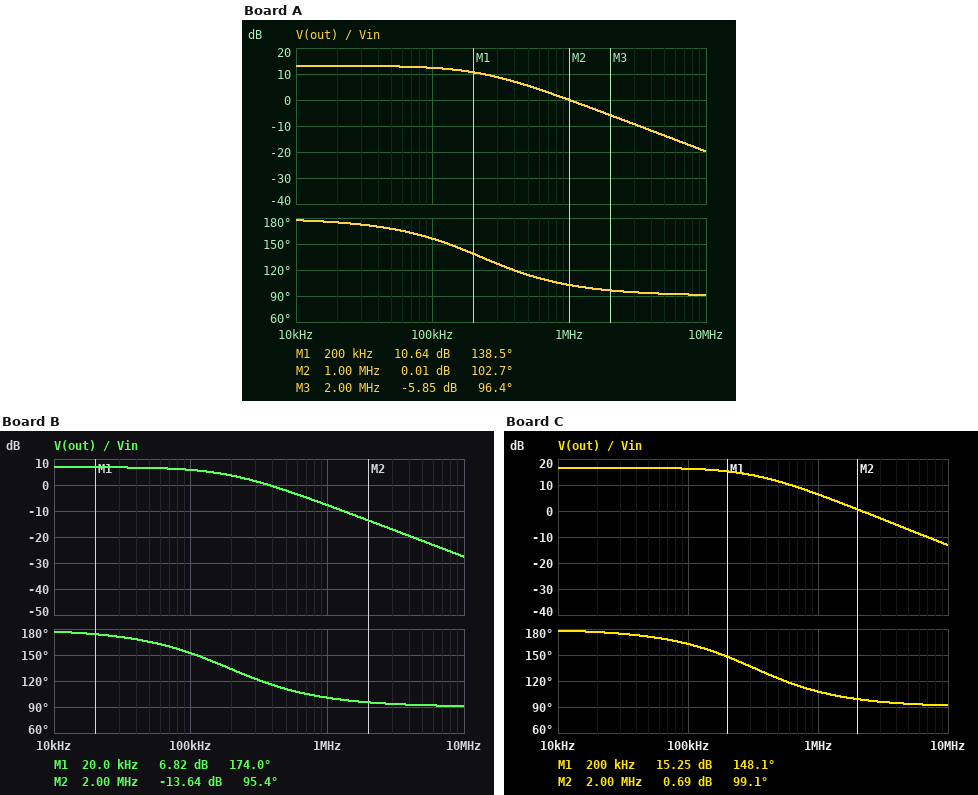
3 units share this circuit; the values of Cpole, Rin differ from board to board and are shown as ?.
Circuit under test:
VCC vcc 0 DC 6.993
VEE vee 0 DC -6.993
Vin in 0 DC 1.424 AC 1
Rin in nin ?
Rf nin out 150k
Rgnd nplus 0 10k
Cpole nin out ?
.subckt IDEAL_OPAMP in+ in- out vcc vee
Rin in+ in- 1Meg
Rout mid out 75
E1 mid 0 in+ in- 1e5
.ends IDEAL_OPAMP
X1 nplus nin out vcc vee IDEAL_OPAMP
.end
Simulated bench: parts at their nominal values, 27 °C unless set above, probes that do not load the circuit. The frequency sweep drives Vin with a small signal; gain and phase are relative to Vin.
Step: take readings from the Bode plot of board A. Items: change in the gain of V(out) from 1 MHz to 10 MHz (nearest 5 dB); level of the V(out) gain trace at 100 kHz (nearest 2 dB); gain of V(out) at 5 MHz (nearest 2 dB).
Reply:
-20 dB
12 dB
-14 dB
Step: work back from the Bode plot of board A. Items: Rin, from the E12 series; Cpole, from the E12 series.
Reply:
33 kΩ
4.7 pF
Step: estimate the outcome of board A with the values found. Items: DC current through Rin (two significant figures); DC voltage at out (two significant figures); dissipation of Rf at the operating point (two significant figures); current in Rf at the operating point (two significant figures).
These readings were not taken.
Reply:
43 µA
-6.5 V
280 µW
43 µA
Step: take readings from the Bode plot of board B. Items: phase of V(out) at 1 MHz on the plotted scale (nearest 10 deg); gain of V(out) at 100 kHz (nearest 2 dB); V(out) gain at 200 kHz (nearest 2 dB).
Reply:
100 deg
6 dB
4 dB
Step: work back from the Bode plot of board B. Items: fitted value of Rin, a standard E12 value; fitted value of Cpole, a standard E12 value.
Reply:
68 kΩ
5.6 pF
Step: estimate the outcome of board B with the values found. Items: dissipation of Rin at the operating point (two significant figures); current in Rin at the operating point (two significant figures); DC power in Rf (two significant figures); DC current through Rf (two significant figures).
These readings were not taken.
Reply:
30 µW
21 µA
66 µW
21 µA
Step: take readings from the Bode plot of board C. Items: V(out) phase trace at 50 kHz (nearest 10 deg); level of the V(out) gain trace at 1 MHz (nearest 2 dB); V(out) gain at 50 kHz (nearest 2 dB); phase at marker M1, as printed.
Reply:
170 deg
6 dB
16 dB
148.1 deg
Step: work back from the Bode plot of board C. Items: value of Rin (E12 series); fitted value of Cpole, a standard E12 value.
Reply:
22 kΩ
3.3 pF
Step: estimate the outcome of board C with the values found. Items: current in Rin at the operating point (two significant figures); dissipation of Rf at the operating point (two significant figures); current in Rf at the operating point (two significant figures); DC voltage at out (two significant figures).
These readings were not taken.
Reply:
65 µA
630 µW
65 µA
-9.7 V
